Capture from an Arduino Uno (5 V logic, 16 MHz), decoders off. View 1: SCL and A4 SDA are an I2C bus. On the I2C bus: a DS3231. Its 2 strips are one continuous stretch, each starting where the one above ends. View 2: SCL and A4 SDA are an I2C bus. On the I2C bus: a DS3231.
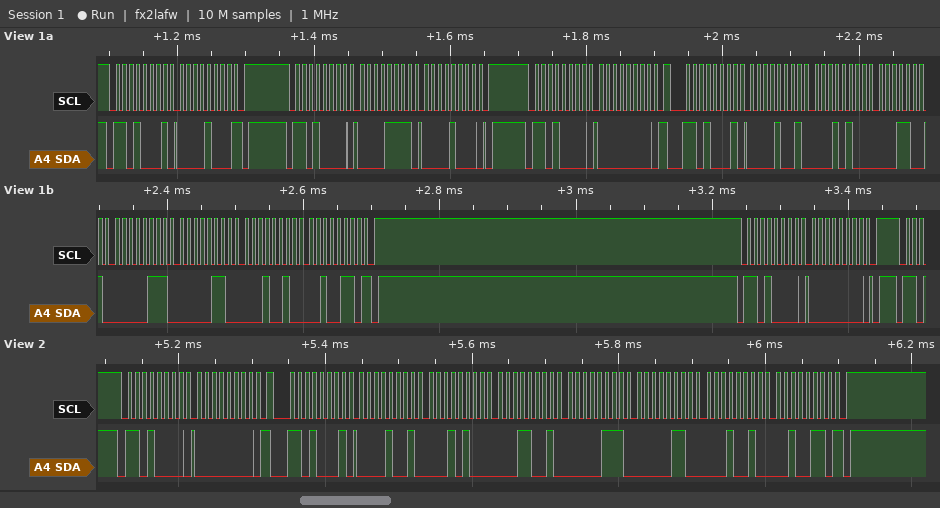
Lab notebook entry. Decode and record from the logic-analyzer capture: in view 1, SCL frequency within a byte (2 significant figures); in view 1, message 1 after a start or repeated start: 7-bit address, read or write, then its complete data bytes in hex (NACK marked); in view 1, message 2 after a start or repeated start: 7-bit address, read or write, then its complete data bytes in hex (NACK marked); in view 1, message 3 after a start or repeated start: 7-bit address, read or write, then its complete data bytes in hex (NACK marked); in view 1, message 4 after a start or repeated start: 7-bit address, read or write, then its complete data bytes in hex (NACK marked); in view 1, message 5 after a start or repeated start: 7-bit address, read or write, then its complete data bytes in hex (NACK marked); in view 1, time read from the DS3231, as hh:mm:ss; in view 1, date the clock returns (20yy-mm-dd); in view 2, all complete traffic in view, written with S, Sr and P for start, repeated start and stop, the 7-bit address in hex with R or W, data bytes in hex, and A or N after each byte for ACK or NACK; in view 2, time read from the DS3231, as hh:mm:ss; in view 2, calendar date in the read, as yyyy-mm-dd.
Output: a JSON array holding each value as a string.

["100 kHz", "0x68 read: 08 NACK", "0x68 write: 0F 08", "0x68 write: 00", "0x68 read: 09 14 19 07 06 12 26 NACK", "0x68 write: 00", "19:14:09", "2026-12-06", "S 68W A 00 A Sr 68R A 09 A 14 A 19 A 07 A 06 A 12 A 26 N P", "19:14:09", "2026-12-06"]
